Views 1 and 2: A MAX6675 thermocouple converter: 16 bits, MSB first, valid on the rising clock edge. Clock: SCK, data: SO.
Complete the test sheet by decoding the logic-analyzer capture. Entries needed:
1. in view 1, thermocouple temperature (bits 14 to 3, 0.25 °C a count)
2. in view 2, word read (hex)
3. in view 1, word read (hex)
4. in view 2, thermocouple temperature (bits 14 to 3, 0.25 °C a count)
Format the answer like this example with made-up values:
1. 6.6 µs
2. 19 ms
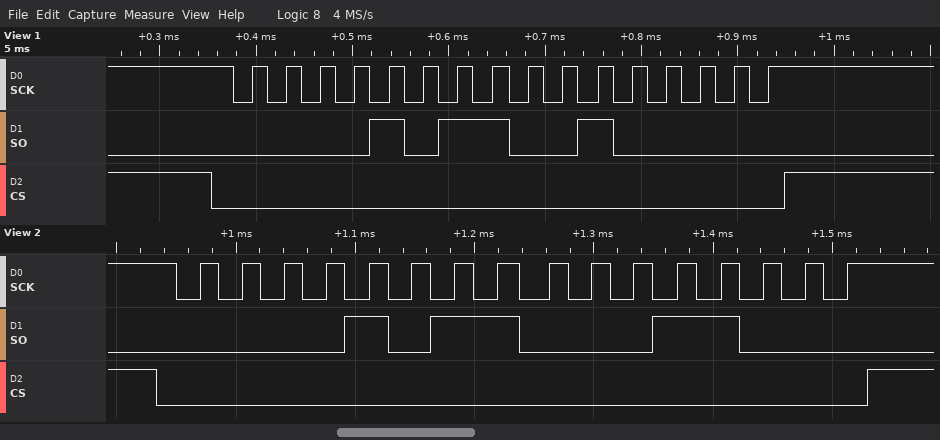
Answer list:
1. 89.00 °C
2. 0x0B18
3. 0x0B20
4. 88.75 °C
